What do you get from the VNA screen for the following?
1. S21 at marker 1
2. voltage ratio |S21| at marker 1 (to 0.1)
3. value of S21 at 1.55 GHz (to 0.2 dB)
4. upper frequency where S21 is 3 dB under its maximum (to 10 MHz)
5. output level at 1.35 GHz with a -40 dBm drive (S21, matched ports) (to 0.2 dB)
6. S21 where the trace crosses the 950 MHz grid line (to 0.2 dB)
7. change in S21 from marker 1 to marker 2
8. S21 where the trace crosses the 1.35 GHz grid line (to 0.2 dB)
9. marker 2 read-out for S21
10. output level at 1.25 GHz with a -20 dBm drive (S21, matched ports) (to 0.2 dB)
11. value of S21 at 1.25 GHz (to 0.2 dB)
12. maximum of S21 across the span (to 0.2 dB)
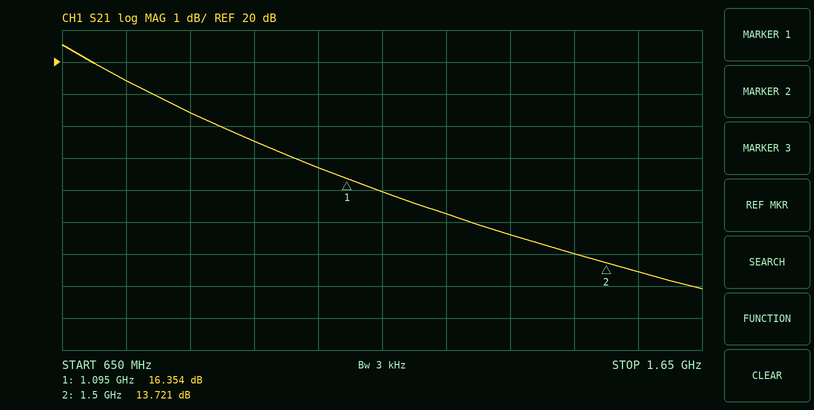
16.354 dB
6.6
13.4 dB
950 MHz
-25.4 dBm
17.6 dB
-2.633 dB
14.6 dB
13.721 dB
-4.8 dBm
15.2 dB
20.6 dB
